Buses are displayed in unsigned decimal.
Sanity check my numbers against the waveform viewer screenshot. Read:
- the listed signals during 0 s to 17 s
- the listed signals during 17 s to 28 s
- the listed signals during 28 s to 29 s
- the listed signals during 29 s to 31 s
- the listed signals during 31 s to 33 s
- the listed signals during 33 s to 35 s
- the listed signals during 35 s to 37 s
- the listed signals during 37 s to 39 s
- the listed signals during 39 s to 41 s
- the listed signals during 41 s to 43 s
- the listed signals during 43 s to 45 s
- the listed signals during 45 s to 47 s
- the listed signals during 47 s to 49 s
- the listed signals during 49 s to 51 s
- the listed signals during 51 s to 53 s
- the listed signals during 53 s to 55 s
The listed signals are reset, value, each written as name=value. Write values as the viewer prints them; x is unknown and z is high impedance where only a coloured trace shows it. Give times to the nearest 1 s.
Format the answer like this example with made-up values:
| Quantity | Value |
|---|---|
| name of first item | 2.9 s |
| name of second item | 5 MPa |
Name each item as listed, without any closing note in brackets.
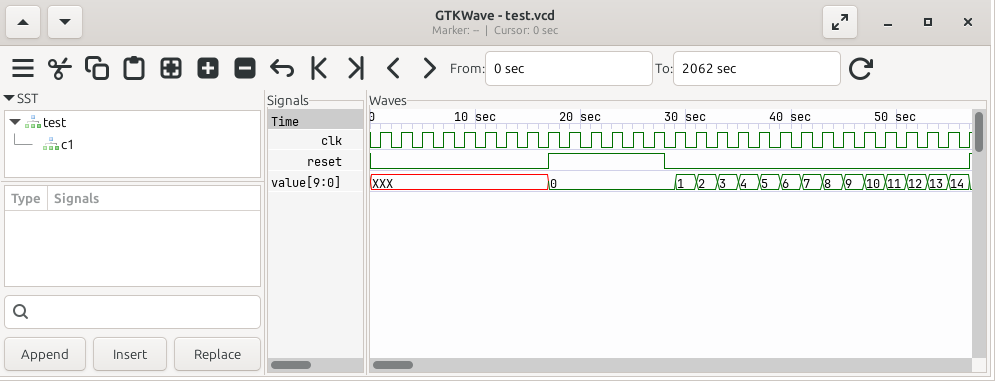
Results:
| Quantity | Value |
|---|---|
| the listed signals during 0 s to 17 s | reset=0, value=XXX |
| the listed signals during 17 s to 28 s | reset=1, value=0 |
| the listed signals during 28 s to 29 s | reset=0, value=0 |
| the listed signals during 29 s to 31 s | reset=0, value=1 |
| the listed signals during 31 s to 33 s | reset=0, value=2 |
| the listed signals during 33 s to 35 s | reset=0, value=3 |
| the listed signals during 35 s to 37 s | reset=0, value=4 |
| the listed signals during 37 s to 39 s | reset=0, value=5 |
| the listed signals during 39 s to 41 s | reset=0, value=6 |
| the listed signals during 41 s to 43 s | reset=0, value=7 |
| the listed signals during 43 s to 45 s | reset=0, value=8 |
| the listed signals during 45 s to 47 s | reset=0, value=9 |
| the listed signals during 47 s to 49 s | reset=0, value=10 |
| the listed signals during 49 s to 51 s | reset=0, value=11 |
| the listed signals during 51 s to 53 s | reset=0, value=12 |
| the listed signals during 53 s to 55 s | reset=0, value=13 |
